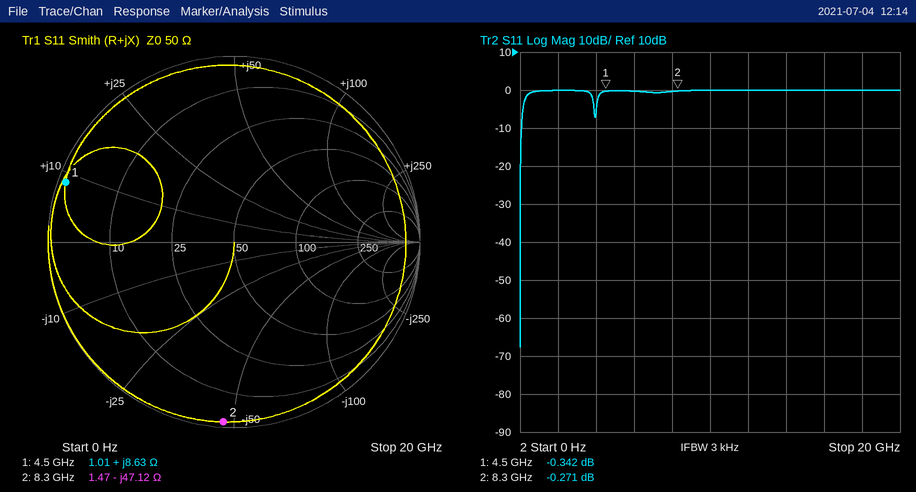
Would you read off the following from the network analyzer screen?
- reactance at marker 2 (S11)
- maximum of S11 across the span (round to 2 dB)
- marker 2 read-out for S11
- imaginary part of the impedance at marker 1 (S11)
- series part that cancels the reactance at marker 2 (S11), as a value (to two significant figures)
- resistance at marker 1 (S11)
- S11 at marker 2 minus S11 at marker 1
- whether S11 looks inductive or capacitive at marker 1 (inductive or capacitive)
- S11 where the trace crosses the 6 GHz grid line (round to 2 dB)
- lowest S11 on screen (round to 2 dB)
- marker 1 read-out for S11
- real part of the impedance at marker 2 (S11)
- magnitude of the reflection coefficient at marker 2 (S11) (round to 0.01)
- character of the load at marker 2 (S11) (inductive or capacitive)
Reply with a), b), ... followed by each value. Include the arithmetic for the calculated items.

a) -47.12 Ω
b) 0 dB
c) -0.271 dB
d) +8.63 Ω
e) L = 47.12 Ω/(2π × 8.3 GHz) ≈ 904 pH, so 900 pH to two significant figures
f) 1.01 Ω
g) -0.271 − (-0.342) = 0.071 dB
h) inductive
i) 0 dB
j) -68 dB
k) -0.342 dB
l) 1.47 Ω
m) 0.97
n) capacitive
